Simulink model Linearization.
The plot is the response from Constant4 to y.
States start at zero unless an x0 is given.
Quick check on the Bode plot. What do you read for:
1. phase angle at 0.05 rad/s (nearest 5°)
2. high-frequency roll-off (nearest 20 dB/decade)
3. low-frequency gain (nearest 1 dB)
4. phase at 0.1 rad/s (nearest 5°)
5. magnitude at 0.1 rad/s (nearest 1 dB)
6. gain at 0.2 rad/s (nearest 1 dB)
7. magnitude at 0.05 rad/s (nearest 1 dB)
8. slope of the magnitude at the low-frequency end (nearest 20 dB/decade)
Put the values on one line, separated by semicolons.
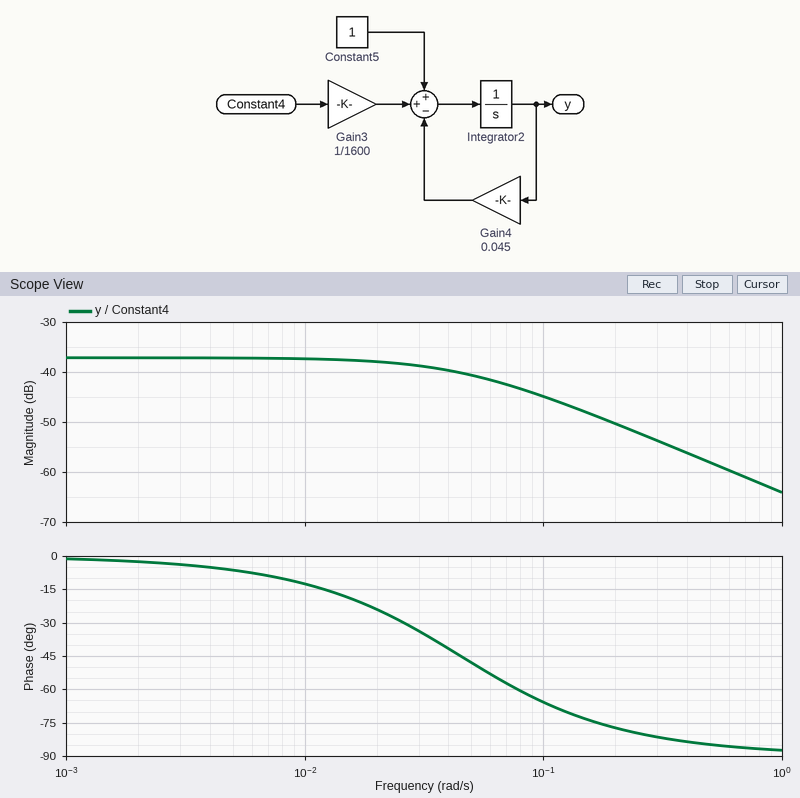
-50°; -20 dB/decade; -37 dB; -65°; -45 dB; -50 dB; -41 dB; 0 dB/decade
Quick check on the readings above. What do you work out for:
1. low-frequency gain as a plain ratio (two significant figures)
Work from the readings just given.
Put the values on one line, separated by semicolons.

0.014
